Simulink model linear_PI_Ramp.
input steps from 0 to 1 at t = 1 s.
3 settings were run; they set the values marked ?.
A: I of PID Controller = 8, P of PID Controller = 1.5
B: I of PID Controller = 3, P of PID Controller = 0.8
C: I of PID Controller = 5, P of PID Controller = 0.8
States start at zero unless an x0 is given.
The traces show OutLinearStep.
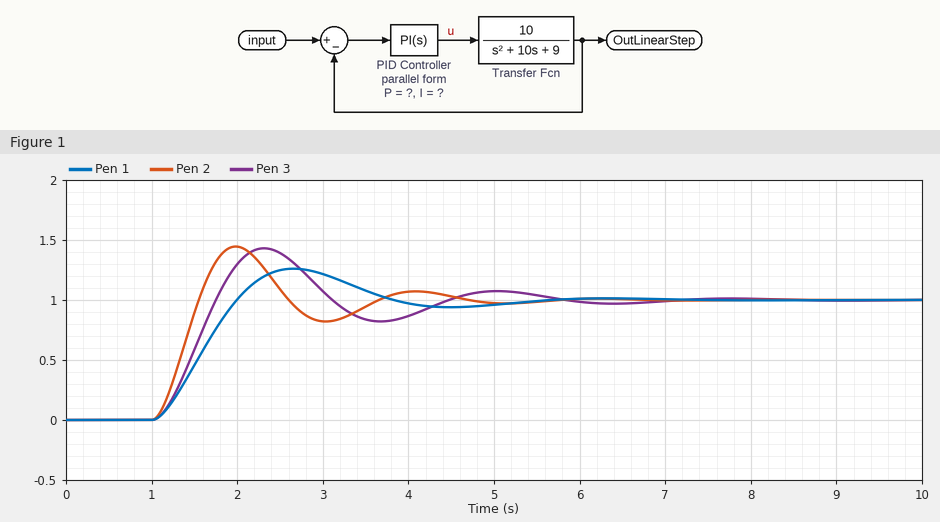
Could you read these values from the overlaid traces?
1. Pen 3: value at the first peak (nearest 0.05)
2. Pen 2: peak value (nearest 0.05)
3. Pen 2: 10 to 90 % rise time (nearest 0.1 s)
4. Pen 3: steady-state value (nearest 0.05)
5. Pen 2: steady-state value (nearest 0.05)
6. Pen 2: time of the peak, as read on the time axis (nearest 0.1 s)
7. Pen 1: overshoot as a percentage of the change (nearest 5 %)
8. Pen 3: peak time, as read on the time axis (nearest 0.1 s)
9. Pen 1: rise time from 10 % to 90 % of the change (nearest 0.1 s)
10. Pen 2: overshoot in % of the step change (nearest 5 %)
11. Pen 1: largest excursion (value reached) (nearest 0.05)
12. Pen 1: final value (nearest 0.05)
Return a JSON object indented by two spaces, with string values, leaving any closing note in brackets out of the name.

{
  "Pen 3: value at the first peak": "1.45",
  "Pen 2: peak value": "1.45",
  "Pen 2: 10 to 90 % rise time": "0.4 s",
  "Pen 3: steady-state value": "1.00",
  "Pen 2: steady-state value": "1.00",
  "Pen 2: time of the peak, as read on the time axis": "2.0 s",
  "Pen 1: overshoot as a percentage of the change": "25 %",
  "Pen 3: peak time, as read on the time axis": "2.3 s",
  "Pen 1: rise time from 10 % to 90 % of the change": "0.7 s",
  "Pen 2: overshoot in % of the step change": "45 %",
  "Pen 1: largest excursion (value reached)": "1.25",
  "Pen 1: final value": "1.00"
}
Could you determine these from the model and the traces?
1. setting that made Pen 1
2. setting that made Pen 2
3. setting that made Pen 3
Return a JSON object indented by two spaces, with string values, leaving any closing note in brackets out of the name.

{
  "setting that made Pen 1": "B",
  "setting that made Pen 2": "A",
  "setting that made Pen 3": "C"
}
